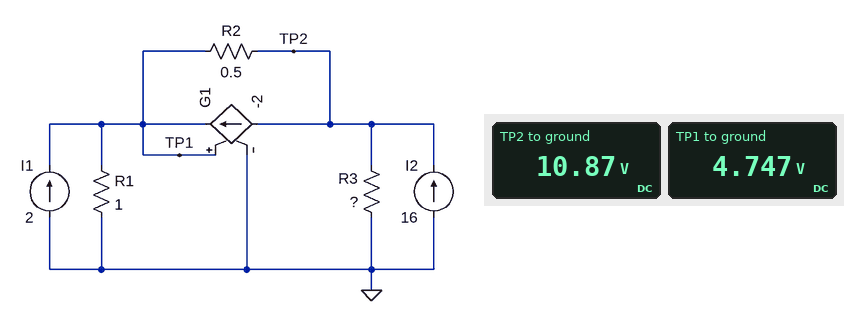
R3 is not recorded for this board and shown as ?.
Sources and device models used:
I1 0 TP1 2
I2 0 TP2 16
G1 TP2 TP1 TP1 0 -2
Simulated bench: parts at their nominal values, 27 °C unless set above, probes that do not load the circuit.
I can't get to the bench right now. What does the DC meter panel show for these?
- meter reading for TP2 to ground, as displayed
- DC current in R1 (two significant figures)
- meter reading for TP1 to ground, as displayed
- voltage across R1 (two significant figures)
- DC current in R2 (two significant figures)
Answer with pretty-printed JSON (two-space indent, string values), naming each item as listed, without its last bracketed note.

{
  "meter reading for TP2 to ground, as displayed": "10.87 V",
  "DC current in R1": "4.7 A",
  "meter reading for TP1 to ground, as displayed": "4.747 V",
  "voltage across R1": "4.7 V",
  "DC current in R2": "12 A"
}
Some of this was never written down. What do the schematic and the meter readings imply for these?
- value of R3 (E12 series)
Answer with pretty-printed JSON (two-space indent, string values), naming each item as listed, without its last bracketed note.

{
  "value of R3": "0.82 Ω"
}
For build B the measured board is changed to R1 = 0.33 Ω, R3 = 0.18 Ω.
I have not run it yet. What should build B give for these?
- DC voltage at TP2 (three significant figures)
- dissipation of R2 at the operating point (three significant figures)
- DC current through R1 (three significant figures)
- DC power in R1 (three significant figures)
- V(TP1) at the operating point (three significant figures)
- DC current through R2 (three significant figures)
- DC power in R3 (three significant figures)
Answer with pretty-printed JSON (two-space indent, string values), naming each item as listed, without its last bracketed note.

{
  "DC voltage at TP2": "2.67 V",
  "dissipation of R2 at the operating point": "5.29 W",
  "DC current through R1": "3.16 A",
  "DC power in R1": "3.30 W",
  "V(TP1) at the operating point": "1.04 V",
  "DC current through R2": "3.25 A",
  "DC power in R3": "39.6 W"
}
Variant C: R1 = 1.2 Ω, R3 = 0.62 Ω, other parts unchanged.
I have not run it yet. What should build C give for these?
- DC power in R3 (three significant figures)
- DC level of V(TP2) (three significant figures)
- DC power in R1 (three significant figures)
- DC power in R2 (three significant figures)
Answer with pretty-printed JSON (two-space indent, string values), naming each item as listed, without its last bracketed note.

{
  "DC power in R3": "131 W",
  "DC level of V(TP2)": "9.02 V",
  "DC power in R1": "14.3 W",
  "DC power in R2": "47.5 W"
}
